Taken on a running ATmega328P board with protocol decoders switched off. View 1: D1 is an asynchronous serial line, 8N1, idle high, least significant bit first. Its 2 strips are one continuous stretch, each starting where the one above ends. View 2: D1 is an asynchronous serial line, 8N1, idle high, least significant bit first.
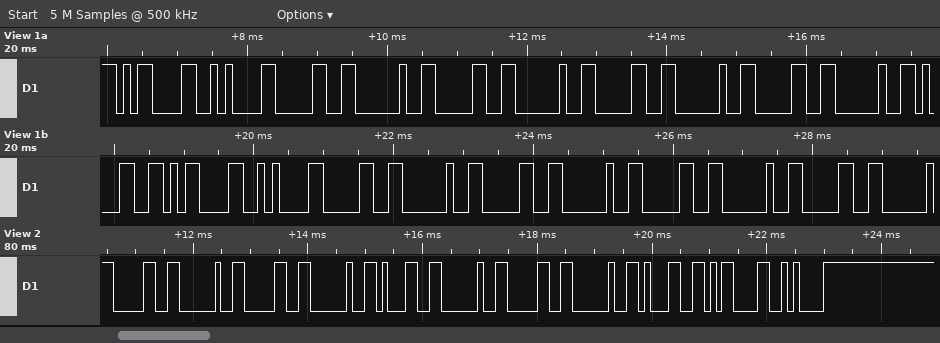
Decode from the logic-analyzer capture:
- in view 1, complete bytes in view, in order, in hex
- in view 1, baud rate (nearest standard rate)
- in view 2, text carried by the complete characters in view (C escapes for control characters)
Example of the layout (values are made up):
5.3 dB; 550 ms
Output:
0D 0A 30 20 30 20 30 20 30 20 31 0D 0A 30 20 30 20 30 20 30; 9600 baud; "0 0 1 0 1\r\n"
